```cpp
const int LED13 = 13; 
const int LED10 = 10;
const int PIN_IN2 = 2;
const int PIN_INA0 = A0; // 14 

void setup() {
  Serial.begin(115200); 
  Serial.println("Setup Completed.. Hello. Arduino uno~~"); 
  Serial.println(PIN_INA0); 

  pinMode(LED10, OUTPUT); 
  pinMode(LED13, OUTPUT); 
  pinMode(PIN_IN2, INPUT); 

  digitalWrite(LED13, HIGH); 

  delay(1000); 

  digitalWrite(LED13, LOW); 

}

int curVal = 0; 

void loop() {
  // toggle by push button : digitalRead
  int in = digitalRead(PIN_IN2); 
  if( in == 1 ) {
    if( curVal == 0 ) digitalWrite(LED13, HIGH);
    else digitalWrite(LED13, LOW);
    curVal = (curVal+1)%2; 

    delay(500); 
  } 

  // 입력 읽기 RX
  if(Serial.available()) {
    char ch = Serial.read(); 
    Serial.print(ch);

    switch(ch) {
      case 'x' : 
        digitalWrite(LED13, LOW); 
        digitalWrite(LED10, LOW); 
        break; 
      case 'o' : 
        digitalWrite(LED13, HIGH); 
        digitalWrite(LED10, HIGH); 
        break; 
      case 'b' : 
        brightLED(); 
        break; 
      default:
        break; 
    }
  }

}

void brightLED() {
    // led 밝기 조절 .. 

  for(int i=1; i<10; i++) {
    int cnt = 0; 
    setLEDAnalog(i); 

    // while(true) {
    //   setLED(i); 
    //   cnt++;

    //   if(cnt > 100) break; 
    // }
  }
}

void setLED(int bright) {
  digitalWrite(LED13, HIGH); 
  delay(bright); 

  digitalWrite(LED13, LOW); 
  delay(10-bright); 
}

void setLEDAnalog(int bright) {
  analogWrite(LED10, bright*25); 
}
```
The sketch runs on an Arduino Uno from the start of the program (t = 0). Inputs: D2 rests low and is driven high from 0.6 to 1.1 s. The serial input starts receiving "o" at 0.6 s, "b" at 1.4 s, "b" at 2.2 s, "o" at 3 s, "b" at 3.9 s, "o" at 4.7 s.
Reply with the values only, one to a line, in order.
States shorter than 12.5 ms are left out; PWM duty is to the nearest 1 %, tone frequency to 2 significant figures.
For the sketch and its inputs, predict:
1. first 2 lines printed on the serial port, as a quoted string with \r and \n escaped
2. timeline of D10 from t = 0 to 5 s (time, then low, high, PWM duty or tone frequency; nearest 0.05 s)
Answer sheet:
"Setup Completed.. Hello. Arduino uno~~\r\n14\r\n"
0 s low; 1.5 s PWM 88 %; 3 s high; 3.9 s PWM 88 %; 4.7 s high
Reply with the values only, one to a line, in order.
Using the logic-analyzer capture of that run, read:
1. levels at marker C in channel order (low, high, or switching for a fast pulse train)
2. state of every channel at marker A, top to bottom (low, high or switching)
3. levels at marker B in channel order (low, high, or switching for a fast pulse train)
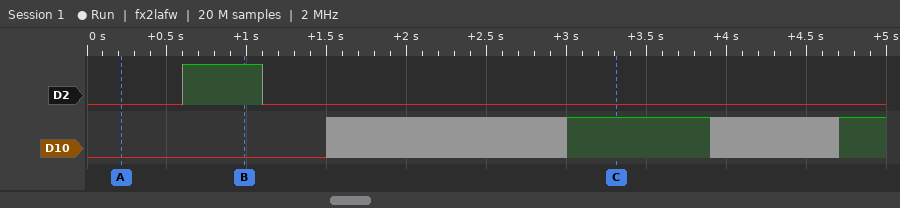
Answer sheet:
D2 low, D10 high
D2 low, D10 low
D2 high, D10 low
